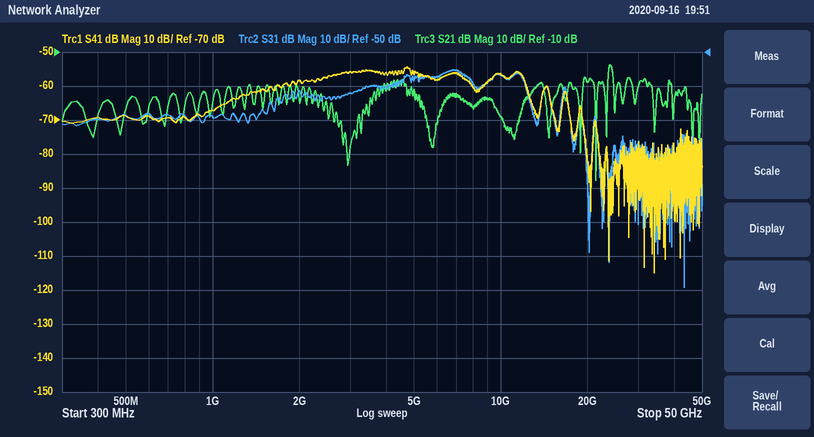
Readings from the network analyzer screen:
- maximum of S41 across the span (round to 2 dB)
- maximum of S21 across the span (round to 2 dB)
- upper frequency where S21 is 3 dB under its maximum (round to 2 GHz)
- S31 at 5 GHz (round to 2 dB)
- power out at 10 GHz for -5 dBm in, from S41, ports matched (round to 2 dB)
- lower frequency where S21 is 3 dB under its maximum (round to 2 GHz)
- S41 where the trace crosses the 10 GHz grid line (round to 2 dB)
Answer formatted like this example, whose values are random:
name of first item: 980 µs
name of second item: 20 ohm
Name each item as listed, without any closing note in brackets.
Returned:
maximum of S41 across the span: -54 dB
maximum of S21 across the span: -14 dB
upper frequency where S21 is 3 dB under its maximum: 24 GHz
S31 at 5 GHz: -58 dB
power out at 10 GHz for -5 dBm in, from S41, ports matched: -62 dBm
lower frequency where S21 is 3 dB under its maximum: 24 GHz
S41 where the trace crosses the 10 GHz grid line: -56 dB
